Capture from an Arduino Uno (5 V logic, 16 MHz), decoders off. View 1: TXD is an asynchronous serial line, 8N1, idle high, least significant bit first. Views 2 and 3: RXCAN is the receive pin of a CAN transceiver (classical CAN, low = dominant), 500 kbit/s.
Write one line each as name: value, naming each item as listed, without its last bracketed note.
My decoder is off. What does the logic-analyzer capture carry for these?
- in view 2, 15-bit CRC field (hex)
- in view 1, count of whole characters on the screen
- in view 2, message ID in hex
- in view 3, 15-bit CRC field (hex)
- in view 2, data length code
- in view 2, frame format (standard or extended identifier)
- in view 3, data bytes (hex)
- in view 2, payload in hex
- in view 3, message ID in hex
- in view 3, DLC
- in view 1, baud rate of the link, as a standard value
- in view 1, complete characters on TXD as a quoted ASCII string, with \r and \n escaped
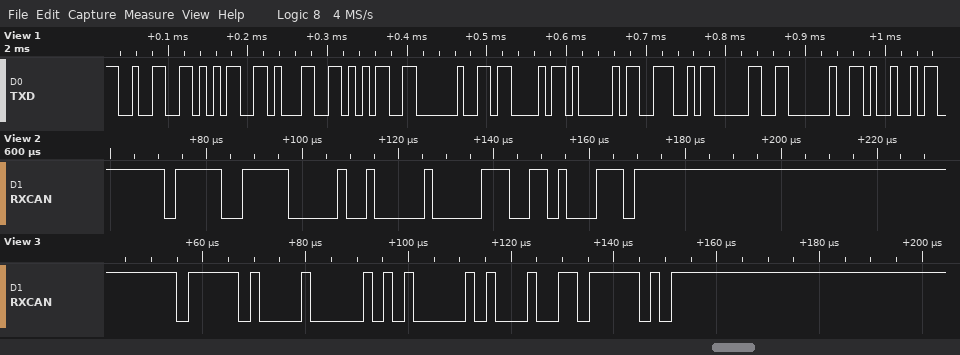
in view 2, 15-bit CRC field: 0x19A3
in view 1, count of whole characters on the screen: 11
in view 2, message ID in hex: 0x7DF
in view 3, 15-bit CRC field: 0x44DF
in view 2, data length code: 1
in view 2, frame format: standard
in view 3, data bytes: 40
in view 2, payload in hex: 00
in view 3, message ID in hex: 0x7E1
in view 3, DLC: 1
in view 1, baud rate of the link, as a standard value: 115200 baud
in view 1, complete characters on TXD as a quoted ASCII string, with \r and \n escaped: "2515 CAN0 I"
